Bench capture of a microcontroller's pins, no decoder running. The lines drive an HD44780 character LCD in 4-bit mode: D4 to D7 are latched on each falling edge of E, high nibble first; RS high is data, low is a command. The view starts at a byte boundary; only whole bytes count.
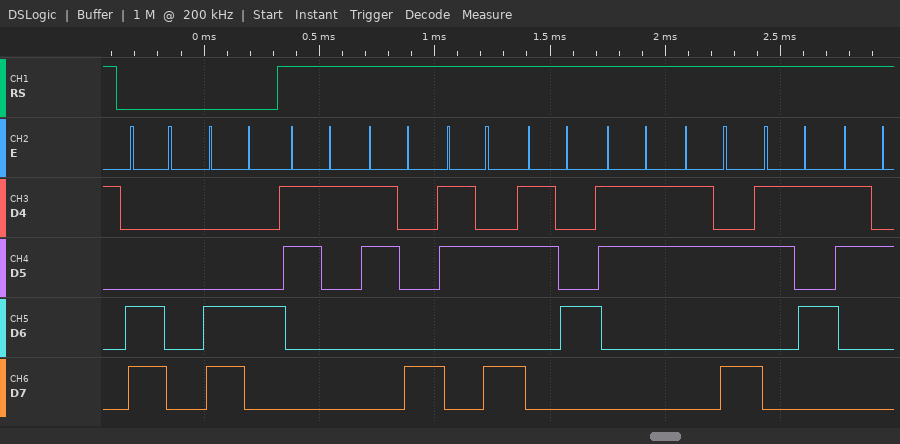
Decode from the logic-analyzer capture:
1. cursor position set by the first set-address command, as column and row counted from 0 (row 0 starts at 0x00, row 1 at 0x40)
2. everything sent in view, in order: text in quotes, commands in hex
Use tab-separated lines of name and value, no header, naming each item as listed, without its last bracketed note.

cursor position set by the first set-address command, as column and row counted from 0	column 0, row 1
everything sent in view, in order: text in quotes, commands in hex	0xC0 0xC4 "18:43:52"
